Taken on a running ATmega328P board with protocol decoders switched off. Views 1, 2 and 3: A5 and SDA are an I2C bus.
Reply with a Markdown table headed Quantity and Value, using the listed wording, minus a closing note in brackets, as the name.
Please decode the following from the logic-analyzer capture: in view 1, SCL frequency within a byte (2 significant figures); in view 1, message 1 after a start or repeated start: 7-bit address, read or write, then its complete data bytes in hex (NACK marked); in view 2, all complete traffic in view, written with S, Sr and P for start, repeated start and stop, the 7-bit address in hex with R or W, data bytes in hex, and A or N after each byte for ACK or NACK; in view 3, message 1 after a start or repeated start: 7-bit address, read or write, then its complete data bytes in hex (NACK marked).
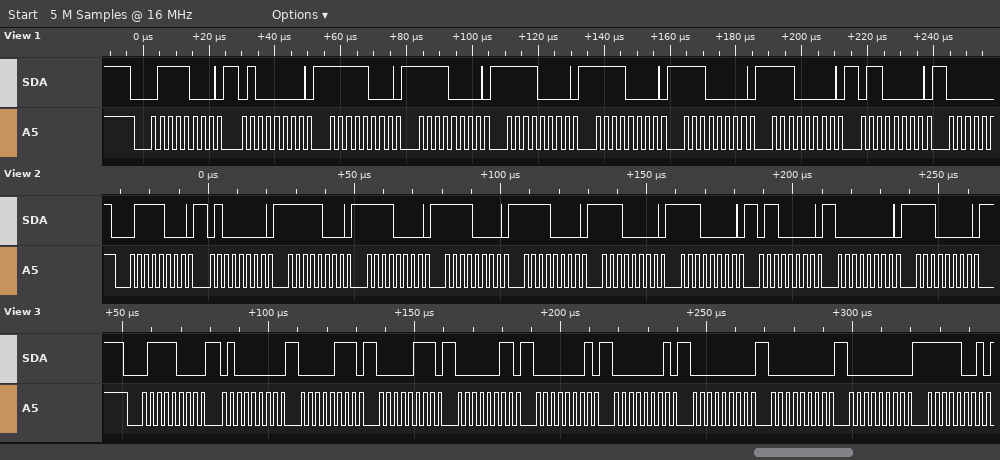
| Quantity | Value |
|---|---|
| in view 1, SCL frequency within a byte | 400 kHz |
| in view 1, message 1 after a start or repeated start: 7-bit address, read or write, then its complete data bytes in hex | 0x3C write: 40 F8 F0 F0 F0 E0 E0 60 |
| in view 2, all complete traffic in view, written with S, Sr and P for start, repeated start and stop, the 7-bit address in hex with R or W, data bytes in hex, and A or N after each byte for ACK or NACK | S 3CW A 40 A F8 A F0 A F0 A F0 A E0 A E0 A 60 A 00 A E0 A |
| in view 3, message 1 after a start or repeated start: 7-bit address, read or write, then its complete data bytes in hex | 0x3C write: 40 07 07 03 01 01 00 00 00 F9 |
